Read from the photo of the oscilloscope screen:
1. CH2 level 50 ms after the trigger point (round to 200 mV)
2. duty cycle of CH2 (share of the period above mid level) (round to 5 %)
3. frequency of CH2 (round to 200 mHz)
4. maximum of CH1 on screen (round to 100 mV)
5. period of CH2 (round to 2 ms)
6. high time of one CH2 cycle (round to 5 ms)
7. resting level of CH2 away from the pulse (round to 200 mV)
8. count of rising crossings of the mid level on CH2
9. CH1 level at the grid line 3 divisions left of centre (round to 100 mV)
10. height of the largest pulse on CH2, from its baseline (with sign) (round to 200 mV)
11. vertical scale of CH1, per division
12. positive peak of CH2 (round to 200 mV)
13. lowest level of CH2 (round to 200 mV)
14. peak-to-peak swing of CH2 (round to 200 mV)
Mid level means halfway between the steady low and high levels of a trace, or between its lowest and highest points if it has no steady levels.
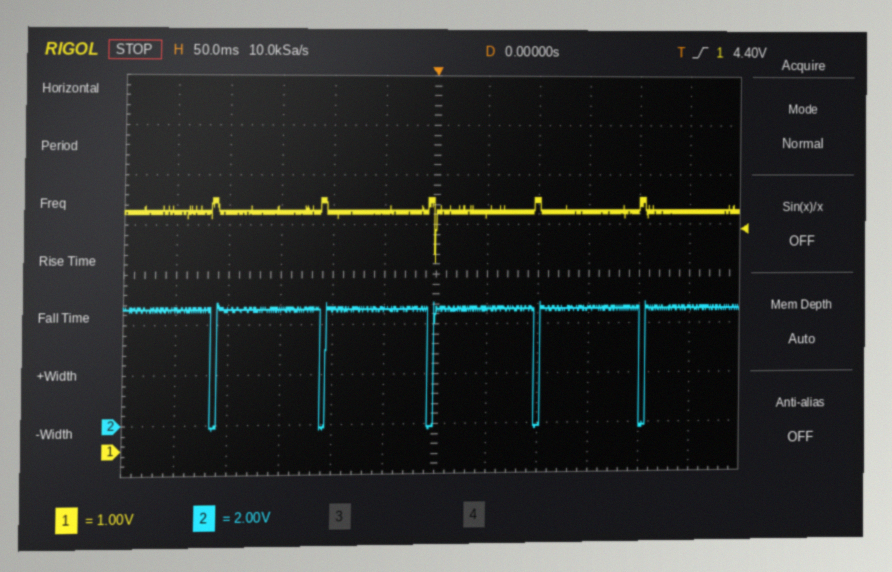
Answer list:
4.6 V
95 %
9.6 Hz
5.0 V
104 ms
100 ms
4.6 V
5
4.8 V
-4.8 V
1 V
4.8 V
-200 mV
5.0 V
